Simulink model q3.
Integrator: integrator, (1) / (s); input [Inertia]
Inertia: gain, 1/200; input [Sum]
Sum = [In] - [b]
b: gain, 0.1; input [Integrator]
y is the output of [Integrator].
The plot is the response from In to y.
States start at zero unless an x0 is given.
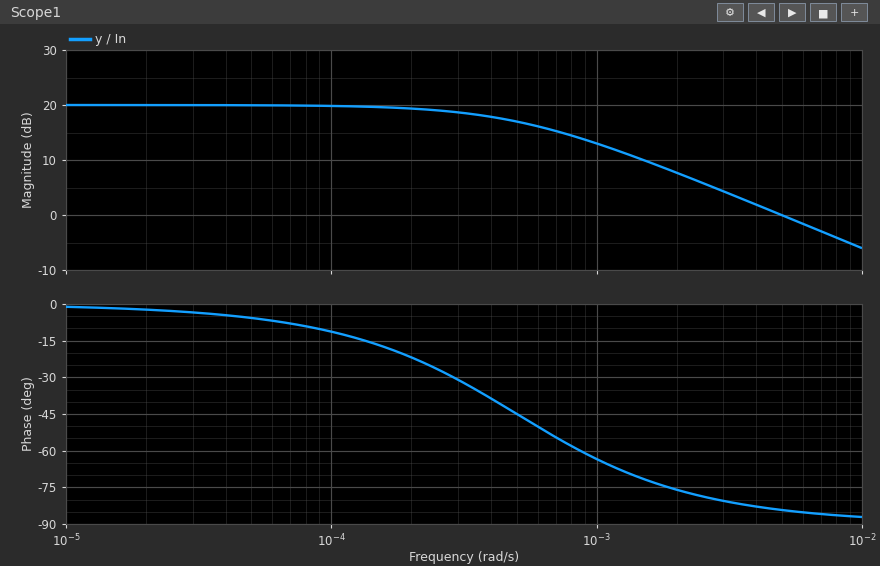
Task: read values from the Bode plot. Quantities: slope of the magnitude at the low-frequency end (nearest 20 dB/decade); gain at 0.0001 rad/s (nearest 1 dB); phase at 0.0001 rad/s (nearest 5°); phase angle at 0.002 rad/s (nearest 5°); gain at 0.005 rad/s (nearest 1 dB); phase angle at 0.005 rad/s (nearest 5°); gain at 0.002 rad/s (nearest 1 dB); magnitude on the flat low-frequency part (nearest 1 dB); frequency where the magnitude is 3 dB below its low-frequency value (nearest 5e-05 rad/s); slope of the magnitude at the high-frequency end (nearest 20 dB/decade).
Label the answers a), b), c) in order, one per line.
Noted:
a) 0 dB/decade
b) 20 dB
c) -10°
d) -75°
e) 0 dB
f) -85°
g) 8 dB
h) 20 dB
i) 0.00050 rad/s
j) -20 dB/decade
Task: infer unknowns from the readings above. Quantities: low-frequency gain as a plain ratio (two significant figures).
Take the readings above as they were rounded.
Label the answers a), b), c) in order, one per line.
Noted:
a) 10
